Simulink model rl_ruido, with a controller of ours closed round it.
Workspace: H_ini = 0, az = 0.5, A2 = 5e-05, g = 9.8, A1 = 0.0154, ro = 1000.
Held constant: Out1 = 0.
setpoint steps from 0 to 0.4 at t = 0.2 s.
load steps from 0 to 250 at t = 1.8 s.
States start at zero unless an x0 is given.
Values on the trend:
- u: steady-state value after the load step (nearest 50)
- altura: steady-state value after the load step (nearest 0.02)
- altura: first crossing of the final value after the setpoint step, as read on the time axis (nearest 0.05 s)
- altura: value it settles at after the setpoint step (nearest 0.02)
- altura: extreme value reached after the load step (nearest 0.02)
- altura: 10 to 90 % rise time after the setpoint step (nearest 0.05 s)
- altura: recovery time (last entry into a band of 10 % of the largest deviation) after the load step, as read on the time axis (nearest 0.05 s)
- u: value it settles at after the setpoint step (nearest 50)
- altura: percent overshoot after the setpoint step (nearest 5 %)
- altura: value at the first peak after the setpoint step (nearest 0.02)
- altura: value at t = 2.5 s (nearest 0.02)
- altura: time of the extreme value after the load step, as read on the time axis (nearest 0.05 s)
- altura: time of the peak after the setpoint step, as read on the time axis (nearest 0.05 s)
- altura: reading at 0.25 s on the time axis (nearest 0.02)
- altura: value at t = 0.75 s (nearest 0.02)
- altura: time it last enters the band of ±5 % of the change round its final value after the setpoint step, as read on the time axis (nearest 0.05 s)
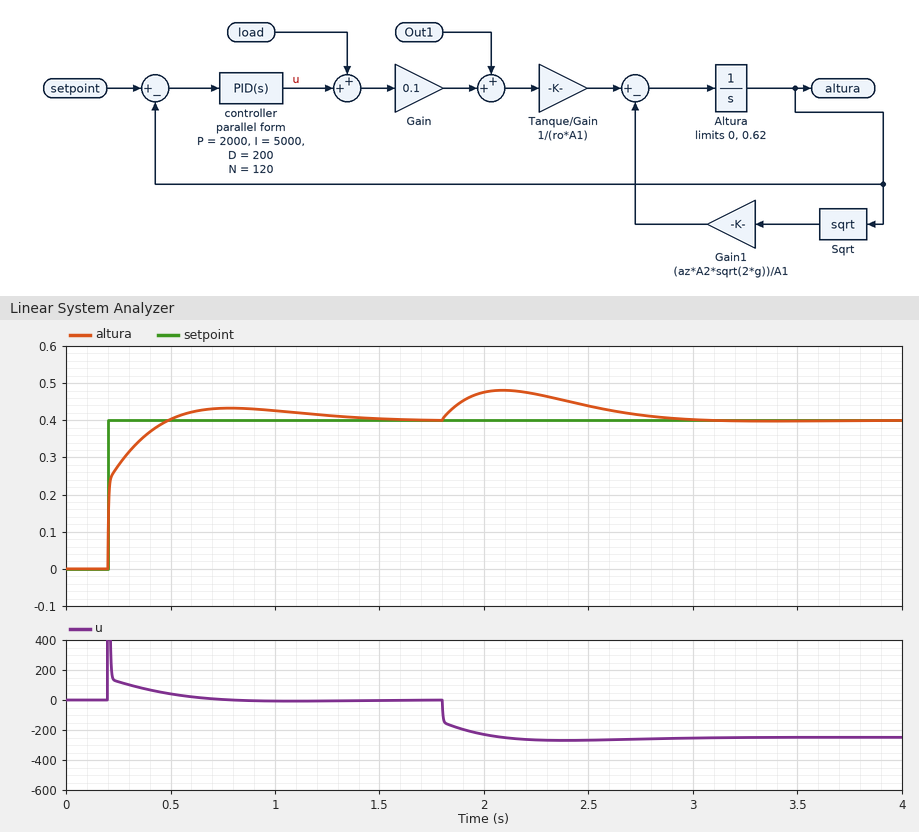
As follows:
-250
0.40
0.50 s
0.40
0.48
0.20 s
2.85 s
0
10 %
0.44
0.44
2.10 s
0.80 s
0.28
0.44
1.10 s
